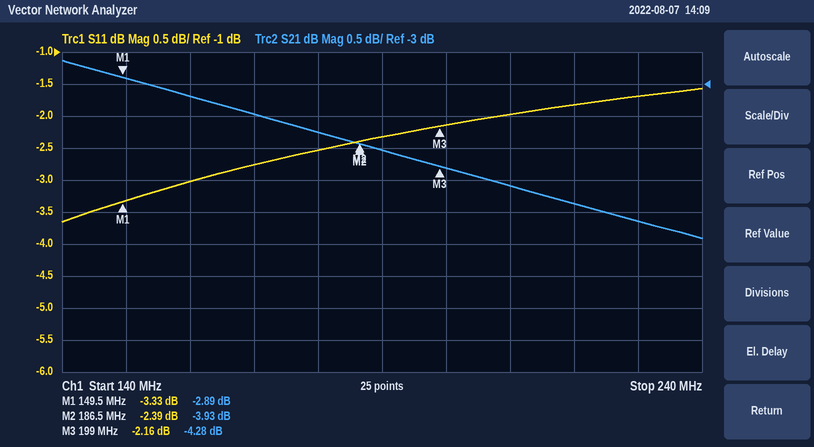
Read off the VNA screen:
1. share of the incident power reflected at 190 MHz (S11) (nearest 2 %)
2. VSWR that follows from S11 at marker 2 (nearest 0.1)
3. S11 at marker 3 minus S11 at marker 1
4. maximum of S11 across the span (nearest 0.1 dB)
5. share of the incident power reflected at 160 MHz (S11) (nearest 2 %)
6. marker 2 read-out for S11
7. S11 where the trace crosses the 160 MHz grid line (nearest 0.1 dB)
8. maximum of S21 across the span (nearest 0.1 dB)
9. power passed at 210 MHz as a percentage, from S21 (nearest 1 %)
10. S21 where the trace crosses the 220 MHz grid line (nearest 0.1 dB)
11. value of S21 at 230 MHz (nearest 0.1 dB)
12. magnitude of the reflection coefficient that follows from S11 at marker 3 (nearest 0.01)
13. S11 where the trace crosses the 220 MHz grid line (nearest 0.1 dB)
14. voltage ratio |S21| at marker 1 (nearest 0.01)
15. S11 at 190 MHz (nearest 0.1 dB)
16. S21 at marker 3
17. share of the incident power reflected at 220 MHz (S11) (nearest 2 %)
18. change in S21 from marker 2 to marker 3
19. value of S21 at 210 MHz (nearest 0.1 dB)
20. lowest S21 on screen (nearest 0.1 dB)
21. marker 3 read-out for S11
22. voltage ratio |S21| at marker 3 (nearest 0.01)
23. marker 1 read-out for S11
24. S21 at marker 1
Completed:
58 %
7.3
1.17 dB
-1.6 dB
50 %
-2.39 dB
-3.0 dB
-2.6 dB
35 %
-4.9 dB
-5.1 dB
0.78
-1.8 dB
0.72
-2.3 dB
-4.28 dB
66 %
-0.35 dB
-4.6 dB
-5.4 dB
-2.16 dB
0.61
-3.33 dB
-2.89 dB
